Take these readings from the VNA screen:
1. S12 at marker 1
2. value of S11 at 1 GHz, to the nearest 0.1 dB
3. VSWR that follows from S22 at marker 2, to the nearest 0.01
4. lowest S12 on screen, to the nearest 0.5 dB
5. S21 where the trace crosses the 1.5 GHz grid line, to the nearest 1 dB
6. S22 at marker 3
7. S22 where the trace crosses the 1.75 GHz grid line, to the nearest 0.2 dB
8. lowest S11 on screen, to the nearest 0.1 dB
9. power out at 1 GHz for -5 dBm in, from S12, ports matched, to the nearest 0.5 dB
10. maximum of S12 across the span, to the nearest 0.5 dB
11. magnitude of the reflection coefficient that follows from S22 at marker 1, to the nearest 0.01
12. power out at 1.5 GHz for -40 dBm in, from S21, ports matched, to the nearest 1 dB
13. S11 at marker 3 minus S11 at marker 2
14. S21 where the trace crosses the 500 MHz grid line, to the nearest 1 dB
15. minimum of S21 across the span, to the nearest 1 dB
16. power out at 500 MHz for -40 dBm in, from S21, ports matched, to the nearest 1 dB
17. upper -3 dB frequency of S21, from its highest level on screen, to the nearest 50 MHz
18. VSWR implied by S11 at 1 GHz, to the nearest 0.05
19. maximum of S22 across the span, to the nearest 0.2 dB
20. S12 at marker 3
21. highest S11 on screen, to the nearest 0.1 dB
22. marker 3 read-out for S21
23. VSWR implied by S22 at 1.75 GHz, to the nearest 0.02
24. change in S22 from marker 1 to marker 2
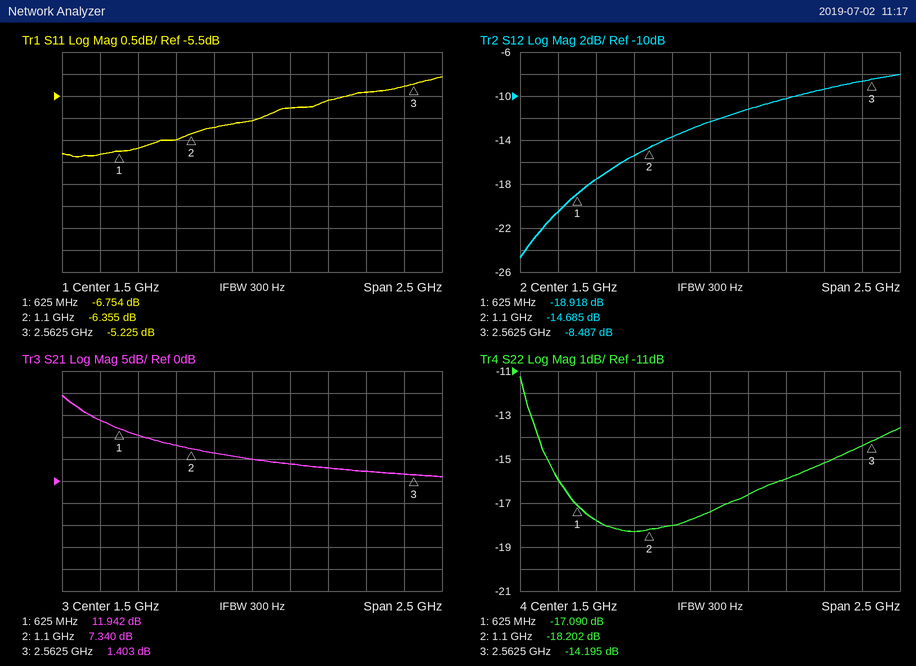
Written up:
-18.918 dB
-6.5 dB
1.28
-24.5 dB
5 dB
-14.195 dB
-16.6 dB
-6.9 dB
-20.5 dBm
-8.0 dB
0.14
-35 dBm
1.130 dB
14 dB
1 dB
-26 dBm
350 MHz
2.80
-11.2 dB
-8.487 dB
-5.1 dB
1.403 dB
1.34
-1.112 dB
